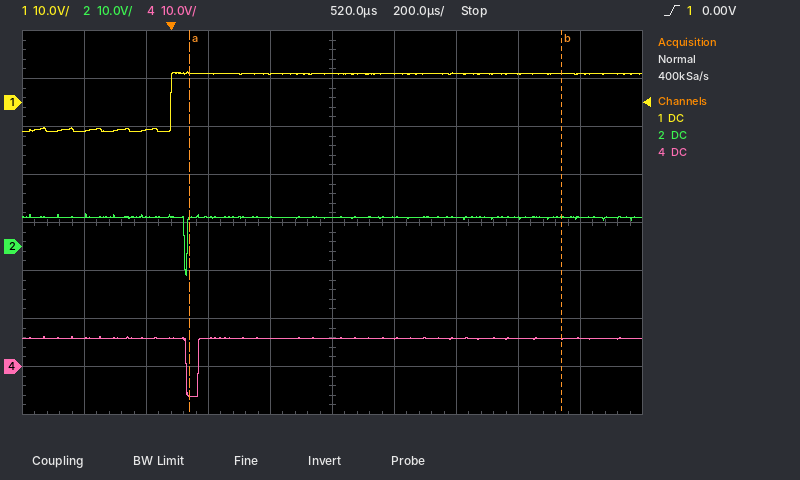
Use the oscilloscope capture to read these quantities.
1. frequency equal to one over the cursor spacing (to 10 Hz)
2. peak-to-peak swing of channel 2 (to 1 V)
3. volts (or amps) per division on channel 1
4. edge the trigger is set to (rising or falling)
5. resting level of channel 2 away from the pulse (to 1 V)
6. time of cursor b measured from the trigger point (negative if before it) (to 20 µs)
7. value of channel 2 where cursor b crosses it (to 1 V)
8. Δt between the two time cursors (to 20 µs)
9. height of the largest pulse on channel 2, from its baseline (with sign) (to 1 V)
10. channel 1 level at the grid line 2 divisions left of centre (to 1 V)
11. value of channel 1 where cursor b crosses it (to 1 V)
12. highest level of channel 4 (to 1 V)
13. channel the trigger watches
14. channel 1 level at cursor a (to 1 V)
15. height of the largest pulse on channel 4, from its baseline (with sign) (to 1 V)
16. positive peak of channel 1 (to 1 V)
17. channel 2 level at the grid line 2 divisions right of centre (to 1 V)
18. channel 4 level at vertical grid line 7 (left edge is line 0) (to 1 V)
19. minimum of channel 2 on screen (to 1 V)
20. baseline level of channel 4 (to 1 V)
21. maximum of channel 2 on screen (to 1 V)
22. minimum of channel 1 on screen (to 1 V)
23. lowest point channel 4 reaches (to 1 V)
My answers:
830 Hz
13 V
10 V
rising
6 V
+1.26 ms
6 V
1.20 ms
-12 V
6 V
6 V
6 V
channel 1
6 V
-12 V
6 V
6 V
6 V
-6 V
6 V
7 V
-6 V
-6 V
